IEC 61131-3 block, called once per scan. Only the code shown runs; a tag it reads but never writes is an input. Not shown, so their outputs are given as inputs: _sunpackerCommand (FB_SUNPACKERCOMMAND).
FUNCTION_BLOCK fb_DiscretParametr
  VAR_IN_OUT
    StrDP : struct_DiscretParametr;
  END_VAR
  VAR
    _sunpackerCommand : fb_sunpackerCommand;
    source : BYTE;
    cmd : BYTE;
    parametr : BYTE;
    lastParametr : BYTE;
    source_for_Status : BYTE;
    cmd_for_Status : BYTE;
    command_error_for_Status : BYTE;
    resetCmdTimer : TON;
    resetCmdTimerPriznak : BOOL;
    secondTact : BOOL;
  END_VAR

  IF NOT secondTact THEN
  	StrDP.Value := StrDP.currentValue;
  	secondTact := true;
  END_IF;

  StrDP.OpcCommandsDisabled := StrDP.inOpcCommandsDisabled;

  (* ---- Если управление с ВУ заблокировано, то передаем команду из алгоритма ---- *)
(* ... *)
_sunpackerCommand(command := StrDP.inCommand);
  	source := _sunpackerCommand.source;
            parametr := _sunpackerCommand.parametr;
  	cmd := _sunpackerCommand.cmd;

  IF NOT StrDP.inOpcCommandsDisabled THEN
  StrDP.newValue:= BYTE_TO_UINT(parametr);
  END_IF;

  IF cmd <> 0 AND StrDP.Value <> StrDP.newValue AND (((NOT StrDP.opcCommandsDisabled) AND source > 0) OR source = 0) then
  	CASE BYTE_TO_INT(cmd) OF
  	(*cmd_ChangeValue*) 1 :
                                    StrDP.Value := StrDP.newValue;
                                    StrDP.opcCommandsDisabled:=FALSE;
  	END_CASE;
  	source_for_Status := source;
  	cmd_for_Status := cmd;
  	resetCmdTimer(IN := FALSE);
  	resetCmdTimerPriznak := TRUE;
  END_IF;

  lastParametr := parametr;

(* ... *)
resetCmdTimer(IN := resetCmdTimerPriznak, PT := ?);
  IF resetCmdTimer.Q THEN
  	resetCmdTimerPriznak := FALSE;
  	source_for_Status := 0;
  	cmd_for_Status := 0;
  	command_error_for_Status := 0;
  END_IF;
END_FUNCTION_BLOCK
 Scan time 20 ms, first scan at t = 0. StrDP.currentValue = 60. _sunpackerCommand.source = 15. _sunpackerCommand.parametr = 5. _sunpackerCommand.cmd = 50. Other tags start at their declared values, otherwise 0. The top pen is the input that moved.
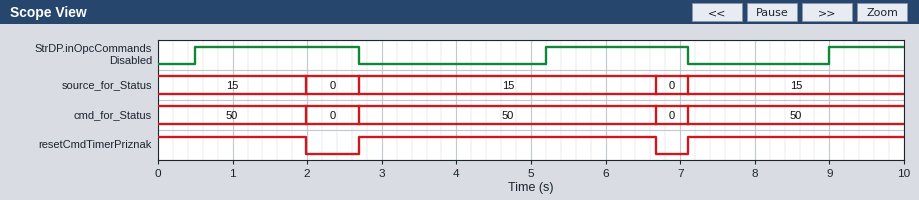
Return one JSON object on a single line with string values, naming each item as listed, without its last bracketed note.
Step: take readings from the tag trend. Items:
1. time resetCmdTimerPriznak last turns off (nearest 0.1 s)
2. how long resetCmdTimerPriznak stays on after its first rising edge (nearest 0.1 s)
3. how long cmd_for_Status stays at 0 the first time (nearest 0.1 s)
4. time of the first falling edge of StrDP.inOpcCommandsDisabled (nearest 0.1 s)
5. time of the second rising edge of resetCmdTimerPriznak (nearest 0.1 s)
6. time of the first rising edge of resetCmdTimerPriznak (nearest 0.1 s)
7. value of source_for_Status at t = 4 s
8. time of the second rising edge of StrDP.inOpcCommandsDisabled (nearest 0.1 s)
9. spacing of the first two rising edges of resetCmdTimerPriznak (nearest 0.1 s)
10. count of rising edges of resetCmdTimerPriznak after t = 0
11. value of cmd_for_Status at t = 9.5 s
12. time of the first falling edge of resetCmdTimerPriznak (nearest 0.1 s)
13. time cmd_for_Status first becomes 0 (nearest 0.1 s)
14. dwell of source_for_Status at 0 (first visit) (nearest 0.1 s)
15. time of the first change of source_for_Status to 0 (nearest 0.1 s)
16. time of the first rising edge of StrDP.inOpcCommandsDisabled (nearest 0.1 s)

{"time resetCmdTimerPriznak last turns off": "6.7 s", "how long resetCmdTimerPriznak stays on after its first rising edge": "4.0 s", "how long cmd_for_Status stays at 0 the first time": "0.7 s", "time of the first falling edge of StrDP.inOpcCommandsDisabled": "2.7 s", "time of the second rising edge of resetCmdTimerPriznak": "7.1 s", "time of the first rising edge of resetCmdTimerPriznak": "2.7 s", "value of source_for_Status at t = 4 s": "15", "time of the second rising edge of StrDP.inOpcCommandsDisabled": "5.2 s", "spacing of the first two rising edges of resetCmdTimerPriznak": "4.4 s", "count of rising edges of resetCmdTimerPriznak after t = 0": "2", "value of cmd_for_Status at t = 9.5 s": "50", "time of the first falling edge of resetCmdTimerPriznak": "2.0 s", "time cmd_for_Status first becomes 0": "2.0 s", "dwell of source_for_Status at 0 (first visit)": "0.7 s", "time of the first change of source_for_Status to 0": "2.0 s", "time of the first rising edge of StrDP.inOpcCommandsDisabled": "0.5 s"}
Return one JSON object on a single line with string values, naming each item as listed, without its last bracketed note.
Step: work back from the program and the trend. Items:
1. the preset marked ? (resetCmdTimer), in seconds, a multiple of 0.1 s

{"the preset marked ? (resetCmdTimer), in seconds, a multiple of 0.1 s": "1.5 s"}
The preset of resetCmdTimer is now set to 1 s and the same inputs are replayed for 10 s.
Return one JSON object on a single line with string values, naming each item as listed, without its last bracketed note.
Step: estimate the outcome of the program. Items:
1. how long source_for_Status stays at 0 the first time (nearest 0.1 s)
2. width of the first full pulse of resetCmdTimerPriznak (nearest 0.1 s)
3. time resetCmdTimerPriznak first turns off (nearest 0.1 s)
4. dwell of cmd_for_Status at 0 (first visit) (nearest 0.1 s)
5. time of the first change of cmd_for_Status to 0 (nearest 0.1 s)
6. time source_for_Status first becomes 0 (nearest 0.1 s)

{"how long source_for_Status stays at 0 the first time": "1.2 s", "width of the first full pulse of resetCmdTimerPriznak": "3.5 s", "time resetCmdTimerPriznak first turns off": "1.5 s", "dwell of cmd_for_Status at 0 (first visit)": "1.2 s", "time of the first change of cmd_for_Status to 0": "1.5 s", "time source_for_Status first becomes 0": "1.5 s"}
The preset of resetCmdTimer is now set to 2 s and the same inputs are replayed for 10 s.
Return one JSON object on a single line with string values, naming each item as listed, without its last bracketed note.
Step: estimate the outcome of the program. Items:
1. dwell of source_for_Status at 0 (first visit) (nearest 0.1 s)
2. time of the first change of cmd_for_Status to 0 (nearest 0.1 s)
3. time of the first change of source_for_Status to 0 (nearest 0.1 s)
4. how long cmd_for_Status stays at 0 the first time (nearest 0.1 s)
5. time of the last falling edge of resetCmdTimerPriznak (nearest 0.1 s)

{"dwell of source_for_Status at 0 (first visit)": "0.2 s", "time of the first change of cmd_for_Status to 0": "2.5 s", "time of the first change of source_for_Status to 0": "2.5 s", "how long cmd_for_Status stays at 0 the first time": "0.2 s", "time of the last falling edge of resetCmdTimerPriznak": "2.5 s"}
